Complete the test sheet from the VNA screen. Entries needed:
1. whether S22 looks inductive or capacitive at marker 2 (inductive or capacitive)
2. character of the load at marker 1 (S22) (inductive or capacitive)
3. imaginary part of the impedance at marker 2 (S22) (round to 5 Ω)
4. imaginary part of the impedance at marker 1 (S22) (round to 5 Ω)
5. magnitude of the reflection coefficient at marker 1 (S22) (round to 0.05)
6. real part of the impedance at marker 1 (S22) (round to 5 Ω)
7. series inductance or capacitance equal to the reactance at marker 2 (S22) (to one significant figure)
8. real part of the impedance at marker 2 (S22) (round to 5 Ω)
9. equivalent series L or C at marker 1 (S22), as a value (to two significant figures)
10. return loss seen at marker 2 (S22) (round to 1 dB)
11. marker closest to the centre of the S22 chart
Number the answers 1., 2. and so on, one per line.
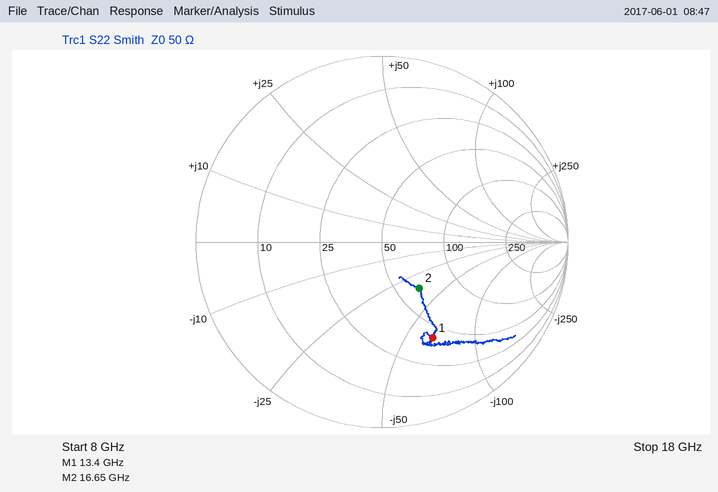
1. capacitive
2. capacitive
3. -35 Ω
4. -65 Ω
5. 0.60
6. 40 Ω
7. 300 fF
8. 65 Ω
9. 180 fF
10. 10 dB
11. marker 2
